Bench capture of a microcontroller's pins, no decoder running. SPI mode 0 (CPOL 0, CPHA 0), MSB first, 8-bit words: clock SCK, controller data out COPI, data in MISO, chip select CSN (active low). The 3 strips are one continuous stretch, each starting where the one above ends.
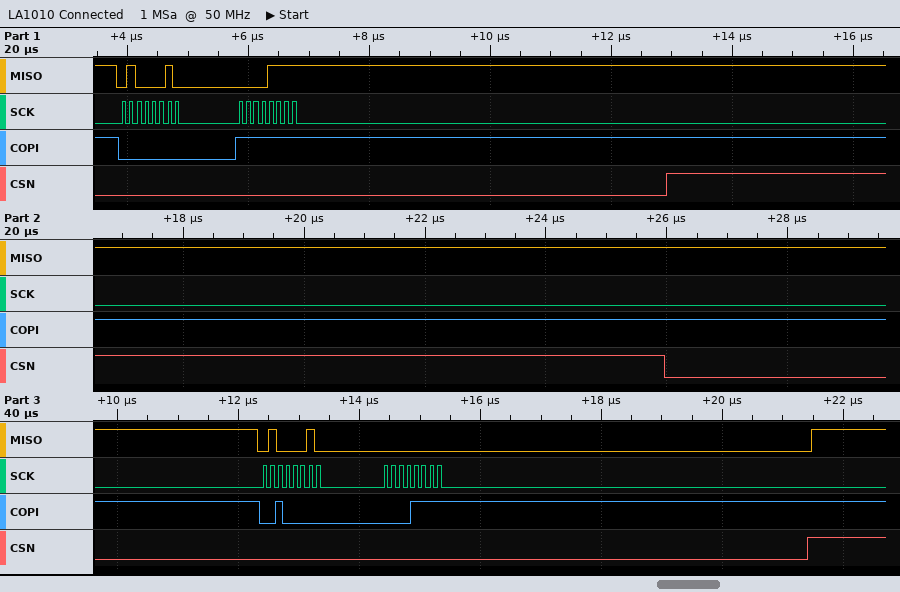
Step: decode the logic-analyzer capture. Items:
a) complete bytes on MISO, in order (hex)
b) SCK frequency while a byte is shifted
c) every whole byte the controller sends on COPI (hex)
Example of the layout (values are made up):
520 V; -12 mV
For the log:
42 0F 42 00; 8 MHz; 00 FF 20 0F
